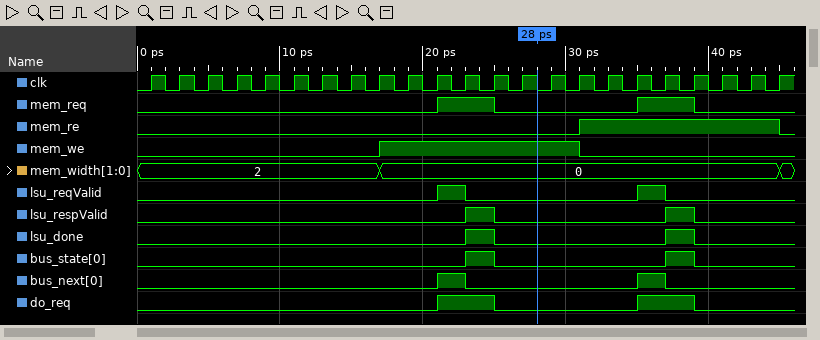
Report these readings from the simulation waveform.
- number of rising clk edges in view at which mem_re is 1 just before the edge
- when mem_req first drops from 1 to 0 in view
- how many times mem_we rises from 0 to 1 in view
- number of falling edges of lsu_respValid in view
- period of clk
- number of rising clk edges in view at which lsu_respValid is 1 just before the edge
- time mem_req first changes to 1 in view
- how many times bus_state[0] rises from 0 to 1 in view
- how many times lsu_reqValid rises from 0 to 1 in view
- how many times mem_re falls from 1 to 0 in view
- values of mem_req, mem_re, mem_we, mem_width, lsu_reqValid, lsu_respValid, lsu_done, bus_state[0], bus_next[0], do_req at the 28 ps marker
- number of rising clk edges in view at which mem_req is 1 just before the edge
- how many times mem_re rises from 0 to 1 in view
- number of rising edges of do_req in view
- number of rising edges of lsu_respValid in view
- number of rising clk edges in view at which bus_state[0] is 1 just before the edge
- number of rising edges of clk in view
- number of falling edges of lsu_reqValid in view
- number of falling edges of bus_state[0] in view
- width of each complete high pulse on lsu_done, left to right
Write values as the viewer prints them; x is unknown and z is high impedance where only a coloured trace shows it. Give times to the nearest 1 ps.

7
25 ps
1
2
2 ps
2
21 ps
2
2
1
mem_req=0, mem_re=0, mem_we=1, mem_width=0, lsu_reqValid=0, lsu_respValid=0, lsu_done=0, bus_state[0]=0, bus_next[0]=0, do_req=0
4
1
2
2
2
23
2
2
2 ps, 2 ps
